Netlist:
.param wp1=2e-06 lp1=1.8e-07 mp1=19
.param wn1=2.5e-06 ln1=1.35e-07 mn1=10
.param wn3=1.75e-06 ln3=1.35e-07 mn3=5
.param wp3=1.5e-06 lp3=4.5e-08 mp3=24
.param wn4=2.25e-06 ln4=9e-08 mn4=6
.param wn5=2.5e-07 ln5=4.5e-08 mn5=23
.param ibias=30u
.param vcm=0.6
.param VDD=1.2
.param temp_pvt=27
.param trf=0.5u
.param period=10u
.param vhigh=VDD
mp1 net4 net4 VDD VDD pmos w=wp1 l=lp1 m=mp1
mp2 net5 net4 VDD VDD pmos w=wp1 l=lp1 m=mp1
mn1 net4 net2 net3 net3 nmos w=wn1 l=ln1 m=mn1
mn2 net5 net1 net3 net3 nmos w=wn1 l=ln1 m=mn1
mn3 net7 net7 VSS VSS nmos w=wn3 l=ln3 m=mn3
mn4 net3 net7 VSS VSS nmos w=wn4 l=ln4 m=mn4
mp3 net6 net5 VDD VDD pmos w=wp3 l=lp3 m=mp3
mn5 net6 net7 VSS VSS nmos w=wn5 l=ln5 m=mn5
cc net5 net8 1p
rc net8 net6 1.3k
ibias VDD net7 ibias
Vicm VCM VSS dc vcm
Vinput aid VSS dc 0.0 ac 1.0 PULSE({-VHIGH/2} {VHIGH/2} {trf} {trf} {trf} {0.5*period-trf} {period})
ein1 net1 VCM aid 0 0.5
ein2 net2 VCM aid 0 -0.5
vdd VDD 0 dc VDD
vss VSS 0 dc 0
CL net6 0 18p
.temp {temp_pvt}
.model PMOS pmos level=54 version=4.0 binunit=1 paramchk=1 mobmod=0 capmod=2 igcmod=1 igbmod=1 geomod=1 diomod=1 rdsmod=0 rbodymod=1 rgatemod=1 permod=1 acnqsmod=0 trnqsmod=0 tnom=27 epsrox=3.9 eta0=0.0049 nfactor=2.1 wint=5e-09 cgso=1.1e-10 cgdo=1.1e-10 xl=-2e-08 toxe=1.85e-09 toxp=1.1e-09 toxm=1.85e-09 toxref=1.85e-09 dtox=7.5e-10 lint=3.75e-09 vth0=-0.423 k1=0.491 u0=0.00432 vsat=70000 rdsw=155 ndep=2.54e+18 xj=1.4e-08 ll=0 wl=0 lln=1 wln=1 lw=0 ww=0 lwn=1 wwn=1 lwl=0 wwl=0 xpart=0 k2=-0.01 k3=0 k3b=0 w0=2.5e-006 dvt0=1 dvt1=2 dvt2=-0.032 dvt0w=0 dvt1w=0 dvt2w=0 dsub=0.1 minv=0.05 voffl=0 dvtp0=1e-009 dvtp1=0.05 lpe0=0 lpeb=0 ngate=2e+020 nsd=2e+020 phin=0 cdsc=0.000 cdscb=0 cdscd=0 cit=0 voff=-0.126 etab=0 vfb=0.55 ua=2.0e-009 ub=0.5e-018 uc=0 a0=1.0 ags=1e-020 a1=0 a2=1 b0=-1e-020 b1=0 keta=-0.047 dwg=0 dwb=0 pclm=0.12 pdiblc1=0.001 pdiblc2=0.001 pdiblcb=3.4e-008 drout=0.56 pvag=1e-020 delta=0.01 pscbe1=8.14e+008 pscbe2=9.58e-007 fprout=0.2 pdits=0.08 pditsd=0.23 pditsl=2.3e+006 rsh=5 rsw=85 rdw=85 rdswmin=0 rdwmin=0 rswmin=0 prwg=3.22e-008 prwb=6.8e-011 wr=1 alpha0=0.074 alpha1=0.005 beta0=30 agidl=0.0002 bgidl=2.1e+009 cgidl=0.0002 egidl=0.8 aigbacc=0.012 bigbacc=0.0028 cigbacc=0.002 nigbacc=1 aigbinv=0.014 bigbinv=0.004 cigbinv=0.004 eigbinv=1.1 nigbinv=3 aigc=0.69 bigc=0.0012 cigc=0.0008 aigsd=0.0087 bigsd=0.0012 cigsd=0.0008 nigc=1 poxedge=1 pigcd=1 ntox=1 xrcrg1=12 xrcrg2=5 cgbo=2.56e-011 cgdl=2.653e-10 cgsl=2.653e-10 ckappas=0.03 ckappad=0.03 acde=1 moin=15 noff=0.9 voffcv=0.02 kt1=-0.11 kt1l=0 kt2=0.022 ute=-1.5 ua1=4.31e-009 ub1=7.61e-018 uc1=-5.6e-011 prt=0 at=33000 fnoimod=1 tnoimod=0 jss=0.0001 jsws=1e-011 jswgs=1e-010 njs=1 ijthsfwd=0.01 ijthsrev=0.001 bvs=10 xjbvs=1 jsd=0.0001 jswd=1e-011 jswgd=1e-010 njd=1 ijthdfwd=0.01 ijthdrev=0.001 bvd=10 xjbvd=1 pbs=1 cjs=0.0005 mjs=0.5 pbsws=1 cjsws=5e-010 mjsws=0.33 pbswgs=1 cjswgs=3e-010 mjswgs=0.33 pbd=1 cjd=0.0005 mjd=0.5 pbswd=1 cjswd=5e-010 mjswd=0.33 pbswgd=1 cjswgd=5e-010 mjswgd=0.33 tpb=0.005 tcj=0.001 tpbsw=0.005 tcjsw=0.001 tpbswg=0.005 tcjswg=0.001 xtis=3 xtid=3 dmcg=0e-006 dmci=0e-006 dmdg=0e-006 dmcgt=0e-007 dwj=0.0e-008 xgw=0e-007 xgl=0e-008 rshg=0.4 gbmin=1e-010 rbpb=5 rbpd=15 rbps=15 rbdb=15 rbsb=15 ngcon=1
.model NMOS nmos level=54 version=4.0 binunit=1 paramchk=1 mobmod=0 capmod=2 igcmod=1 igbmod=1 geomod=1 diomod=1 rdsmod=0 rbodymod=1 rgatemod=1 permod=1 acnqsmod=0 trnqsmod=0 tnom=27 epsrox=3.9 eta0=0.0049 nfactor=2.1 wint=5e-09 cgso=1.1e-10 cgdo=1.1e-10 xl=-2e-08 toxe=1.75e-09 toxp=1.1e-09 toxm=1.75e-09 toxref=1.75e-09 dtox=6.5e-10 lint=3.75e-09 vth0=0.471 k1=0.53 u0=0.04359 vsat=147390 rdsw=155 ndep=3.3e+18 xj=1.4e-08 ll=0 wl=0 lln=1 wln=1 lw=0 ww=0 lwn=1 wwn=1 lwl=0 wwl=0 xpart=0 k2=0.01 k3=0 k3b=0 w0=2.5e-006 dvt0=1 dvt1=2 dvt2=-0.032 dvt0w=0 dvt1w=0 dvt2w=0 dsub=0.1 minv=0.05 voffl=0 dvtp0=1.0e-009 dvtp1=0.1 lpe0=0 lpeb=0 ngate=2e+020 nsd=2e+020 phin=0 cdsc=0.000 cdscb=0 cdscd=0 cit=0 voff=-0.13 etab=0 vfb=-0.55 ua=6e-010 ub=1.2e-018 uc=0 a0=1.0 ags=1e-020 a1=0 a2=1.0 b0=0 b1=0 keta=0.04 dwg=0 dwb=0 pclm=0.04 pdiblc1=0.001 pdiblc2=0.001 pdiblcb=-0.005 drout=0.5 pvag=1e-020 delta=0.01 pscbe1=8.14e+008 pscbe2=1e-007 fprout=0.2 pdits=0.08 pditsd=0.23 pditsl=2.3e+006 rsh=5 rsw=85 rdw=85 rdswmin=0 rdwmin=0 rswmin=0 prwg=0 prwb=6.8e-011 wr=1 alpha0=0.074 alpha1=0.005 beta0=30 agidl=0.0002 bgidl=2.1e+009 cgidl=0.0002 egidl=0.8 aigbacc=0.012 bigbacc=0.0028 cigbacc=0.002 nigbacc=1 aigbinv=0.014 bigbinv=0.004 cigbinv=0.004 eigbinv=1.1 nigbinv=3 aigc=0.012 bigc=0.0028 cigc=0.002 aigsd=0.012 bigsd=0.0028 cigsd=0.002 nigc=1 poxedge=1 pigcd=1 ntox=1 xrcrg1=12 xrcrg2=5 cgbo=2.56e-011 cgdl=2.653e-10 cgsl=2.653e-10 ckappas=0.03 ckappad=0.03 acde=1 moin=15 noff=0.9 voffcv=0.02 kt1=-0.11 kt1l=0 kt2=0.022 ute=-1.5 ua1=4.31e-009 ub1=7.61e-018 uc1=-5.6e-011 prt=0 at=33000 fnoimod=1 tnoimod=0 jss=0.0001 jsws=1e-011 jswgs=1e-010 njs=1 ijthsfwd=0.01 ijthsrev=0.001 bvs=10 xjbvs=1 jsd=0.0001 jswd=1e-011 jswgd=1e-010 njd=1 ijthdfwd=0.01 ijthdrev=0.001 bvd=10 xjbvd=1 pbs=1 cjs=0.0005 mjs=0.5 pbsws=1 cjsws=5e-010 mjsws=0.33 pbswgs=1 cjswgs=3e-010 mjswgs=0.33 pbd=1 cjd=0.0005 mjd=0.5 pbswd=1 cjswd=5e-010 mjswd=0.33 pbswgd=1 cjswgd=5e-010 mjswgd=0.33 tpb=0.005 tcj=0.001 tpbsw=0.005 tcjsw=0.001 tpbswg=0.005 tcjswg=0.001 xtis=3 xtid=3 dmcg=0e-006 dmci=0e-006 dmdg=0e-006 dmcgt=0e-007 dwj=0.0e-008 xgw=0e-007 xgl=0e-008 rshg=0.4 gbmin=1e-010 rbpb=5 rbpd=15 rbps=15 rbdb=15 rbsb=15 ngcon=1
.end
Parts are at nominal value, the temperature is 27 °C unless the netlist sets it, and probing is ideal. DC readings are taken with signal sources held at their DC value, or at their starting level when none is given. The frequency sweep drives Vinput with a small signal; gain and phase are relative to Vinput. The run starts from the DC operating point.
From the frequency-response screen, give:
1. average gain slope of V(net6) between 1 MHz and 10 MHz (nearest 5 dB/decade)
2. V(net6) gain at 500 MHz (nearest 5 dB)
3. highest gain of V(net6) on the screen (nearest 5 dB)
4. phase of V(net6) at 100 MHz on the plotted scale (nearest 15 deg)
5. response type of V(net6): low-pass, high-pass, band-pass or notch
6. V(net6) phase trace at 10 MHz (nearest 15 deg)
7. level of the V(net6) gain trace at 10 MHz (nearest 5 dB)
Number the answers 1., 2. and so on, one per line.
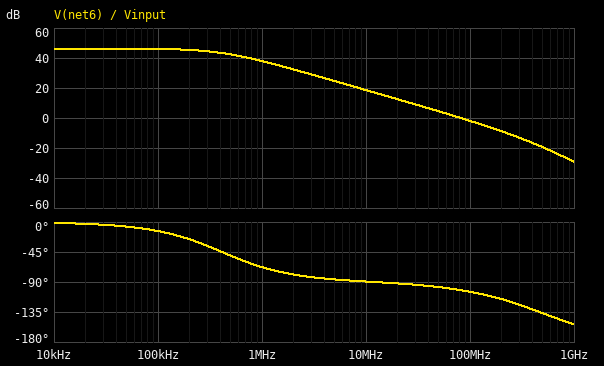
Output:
1. -20 dB/decade
2. -20 dB
3. 45 dB
4. -105 deg
5. low-pass
6. -90 deg
7. 20 dB
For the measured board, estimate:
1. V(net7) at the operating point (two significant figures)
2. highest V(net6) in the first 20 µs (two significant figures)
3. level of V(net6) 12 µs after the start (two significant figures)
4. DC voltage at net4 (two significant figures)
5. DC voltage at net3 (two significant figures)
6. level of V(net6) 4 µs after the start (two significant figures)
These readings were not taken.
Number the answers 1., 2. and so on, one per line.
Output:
1. 420 mV
2. 1.2 V
3. 1.2 V
4. 720 mV
5. 220 mV
6. 1.2 V
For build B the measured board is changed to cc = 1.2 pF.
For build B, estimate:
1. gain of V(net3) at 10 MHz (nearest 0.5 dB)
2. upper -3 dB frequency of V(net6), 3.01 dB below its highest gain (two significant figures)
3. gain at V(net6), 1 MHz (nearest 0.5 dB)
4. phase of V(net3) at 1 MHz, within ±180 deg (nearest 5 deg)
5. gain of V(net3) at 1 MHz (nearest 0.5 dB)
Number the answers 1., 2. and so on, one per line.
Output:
1. -39.5 dB
2. 350 kHz
3. 36.5 dB
4. 110 deg
5. -20.5 dB
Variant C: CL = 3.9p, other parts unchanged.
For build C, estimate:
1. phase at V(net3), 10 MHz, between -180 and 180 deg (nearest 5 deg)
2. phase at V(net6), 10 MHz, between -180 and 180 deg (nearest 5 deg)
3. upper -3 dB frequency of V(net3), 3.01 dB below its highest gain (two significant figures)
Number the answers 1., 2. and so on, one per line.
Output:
1. 100 deg
2. -85 deg
3. 420 kHz
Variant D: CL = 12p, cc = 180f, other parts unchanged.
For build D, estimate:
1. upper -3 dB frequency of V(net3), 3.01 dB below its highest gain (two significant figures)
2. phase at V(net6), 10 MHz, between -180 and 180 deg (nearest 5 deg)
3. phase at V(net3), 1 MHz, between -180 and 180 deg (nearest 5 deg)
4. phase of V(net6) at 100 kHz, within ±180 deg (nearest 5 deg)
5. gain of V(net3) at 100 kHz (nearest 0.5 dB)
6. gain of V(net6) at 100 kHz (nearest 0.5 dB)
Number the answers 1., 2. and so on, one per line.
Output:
1. 1.9 MHz
2. -85 deg
3. 155 deg
4. -5 deg
5. -10.5 dB
6. 46.5 dB
